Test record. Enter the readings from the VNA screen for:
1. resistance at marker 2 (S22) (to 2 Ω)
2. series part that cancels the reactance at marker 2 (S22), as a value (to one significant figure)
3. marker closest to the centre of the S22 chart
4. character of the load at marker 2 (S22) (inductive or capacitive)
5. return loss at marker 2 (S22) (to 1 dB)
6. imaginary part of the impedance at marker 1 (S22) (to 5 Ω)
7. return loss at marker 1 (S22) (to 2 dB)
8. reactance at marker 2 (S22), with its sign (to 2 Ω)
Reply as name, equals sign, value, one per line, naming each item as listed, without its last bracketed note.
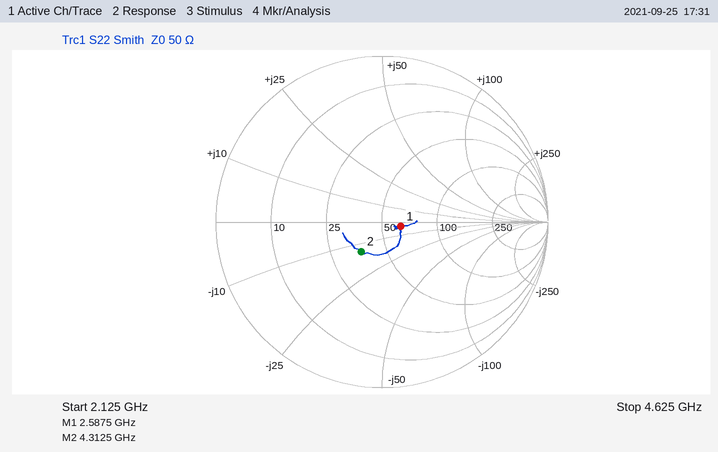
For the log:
resistance at marker 2 (S22) = 36 Ω
series part that cancels the reactance at marker 2 (S22), as a value = 500 pH
marker closest to the centre of the S22 chart = marker 1
character of the load at marker 2 (S22) = capacitive
return loss at marker 2 (S22) = 13 dB
imaginary part of the impedance at marker 1 (S22) = -5 Ω
return loss at marker 1 (S22) = 18 dB
reactance at marker 2 (S22), with its sign = -14 Ω
